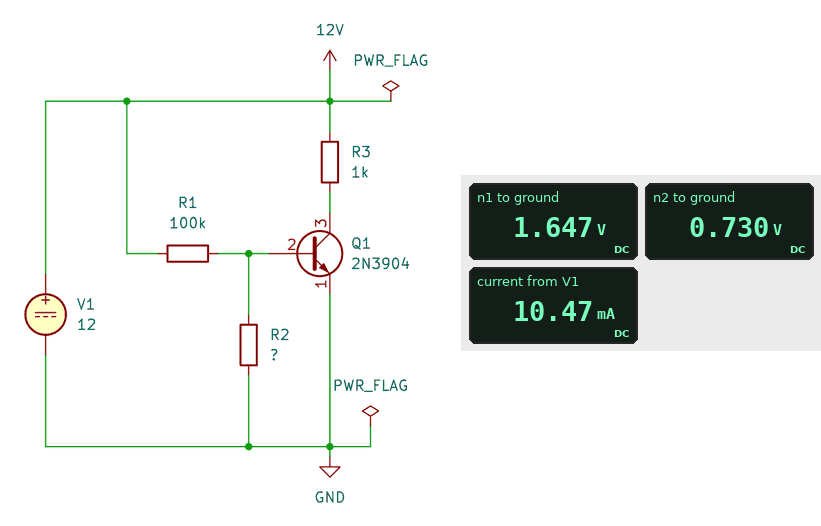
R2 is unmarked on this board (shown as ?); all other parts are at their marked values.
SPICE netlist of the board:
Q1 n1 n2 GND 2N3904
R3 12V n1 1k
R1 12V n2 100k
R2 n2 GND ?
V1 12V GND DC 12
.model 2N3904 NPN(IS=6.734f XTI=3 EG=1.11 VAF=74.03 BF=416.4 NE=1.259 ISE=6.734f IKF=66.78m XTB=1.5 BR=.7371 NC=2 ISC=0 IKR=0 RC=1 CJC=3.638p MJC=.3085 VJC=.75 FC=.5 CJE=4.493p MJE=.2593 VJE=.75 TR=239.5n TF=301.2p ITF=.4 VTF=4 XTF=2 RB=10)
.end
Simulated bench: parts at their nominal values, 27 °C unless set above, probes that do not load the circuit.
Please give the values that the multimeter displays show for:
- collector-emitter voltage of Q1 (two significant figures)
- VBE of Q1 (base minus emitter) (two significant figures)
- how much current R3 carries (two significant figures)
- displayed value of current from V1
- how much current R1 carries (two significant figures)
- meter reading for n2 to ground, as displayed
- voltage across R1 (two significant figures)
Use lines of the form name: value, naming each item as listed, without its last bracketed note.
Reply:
collector-emitter voltage of Q1: 1.6 V
VBE of Q1 (base minus emitter): 730 mV
how much current R3 carries: 10 mA
displayed value of current from V1: 10.47 mA
how much current R1 carries: 110 µA
meter reading for n2 to ground, as displayed: 0.730 V
voltage across R1: 11 V
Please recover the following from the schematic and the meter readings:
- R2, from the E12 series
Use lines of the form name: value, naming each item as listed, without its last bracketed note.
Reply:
R2, from the E12 series: 15 kΩ
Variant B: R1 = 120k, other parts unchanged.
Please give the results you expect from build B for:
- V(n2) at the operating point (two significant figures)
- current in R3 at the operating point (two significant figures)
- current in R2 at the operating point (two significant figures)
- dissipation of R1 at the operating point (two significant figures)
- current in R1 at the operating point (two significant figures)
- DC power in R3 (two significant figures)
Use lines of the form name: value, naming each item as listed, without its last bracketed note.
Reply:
V(n2) at the operating point: 720 mV
current in R3 at the operating point: 7.7 mA
current in R2 at the operating point: 48 µA
dissipation of R1 at the operating point: 1.1 mW
current in R1 at the operating point: 94 µA
DC power in R3: 59 mW
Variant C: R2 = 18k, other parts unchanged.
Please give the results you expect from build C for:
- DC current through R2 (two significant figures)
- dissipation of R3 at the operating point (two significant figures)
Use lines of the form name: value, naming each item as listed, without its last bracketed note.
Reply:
DC current through R2: 41 µA
dissipation of R3 at the operating point: 130 mW
